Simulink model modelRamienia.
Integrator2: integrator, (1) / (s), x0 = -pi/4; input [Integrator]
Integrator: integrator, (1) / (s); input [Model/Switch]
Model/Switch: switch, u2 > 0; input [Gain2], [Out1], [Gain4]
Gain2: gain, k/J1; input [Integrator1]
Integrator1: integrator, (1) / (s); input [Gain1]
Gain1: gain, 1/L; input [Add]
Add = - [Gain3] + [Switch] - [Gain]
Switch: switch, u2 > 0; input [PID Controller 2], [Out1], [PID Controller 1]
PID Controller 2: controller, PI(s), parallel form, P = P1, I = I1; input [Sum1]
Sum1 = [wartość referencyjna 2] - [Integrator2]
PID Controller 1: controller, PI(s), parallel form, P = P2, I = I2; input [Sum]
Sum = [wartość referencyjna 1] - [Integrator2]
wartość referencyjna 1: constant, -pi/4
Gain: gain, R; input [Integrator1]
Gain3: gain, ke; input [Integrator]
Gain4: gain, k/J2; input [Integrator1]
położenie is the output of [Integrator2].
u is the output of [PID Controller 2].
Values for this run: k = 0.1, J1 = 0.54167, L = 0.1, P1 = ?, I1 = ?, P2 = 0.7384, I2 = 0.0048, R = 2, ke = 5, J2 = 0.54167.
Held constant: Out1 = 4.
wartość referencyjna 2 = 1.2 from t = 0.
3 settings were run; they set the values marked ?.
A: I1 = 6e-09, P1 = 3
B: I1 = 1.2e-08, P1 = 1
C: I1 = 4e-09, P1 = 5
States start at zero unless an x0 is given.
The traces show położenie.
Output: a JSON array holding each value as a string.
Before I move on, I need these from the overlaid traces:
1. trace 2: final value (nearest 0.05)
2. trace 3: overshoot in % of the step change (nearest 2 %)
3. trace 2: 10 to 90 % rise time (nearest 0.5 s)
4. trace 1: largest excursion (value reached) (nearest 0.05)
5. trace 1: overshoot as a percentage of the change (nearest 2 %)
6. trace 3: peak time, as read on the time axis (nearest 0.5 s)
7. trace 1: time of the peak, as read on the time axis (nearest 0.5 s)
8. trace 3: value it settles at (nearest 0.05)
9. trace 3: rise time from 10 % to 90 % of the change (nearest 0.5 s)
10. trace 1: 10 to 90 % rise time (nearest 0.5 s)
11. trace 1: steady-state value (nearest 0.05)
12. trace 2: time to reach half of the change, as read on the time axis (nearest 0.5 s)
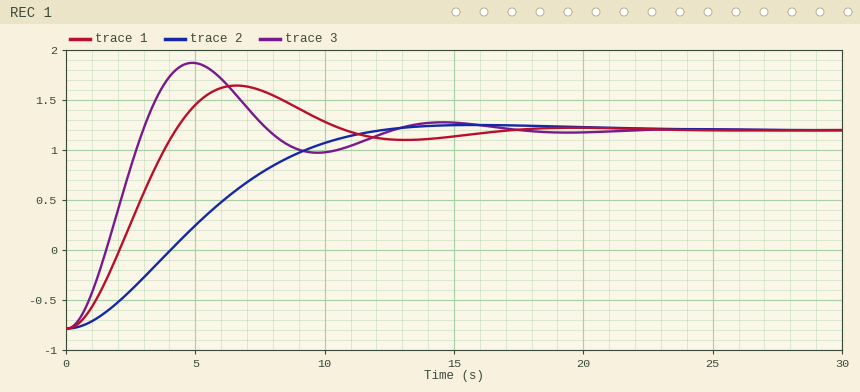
["1.20", "34 %", "7.5 s", "1.65", "22 %", "5.0 s", "6.5 s", "1.20", "2.0 s", "3.0 s", "1.20", "5.0 s"]
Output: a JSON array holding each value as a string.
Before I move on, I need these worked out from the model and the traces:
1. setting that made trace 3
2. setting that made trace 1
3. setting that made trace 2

["C", "A", "B"]
